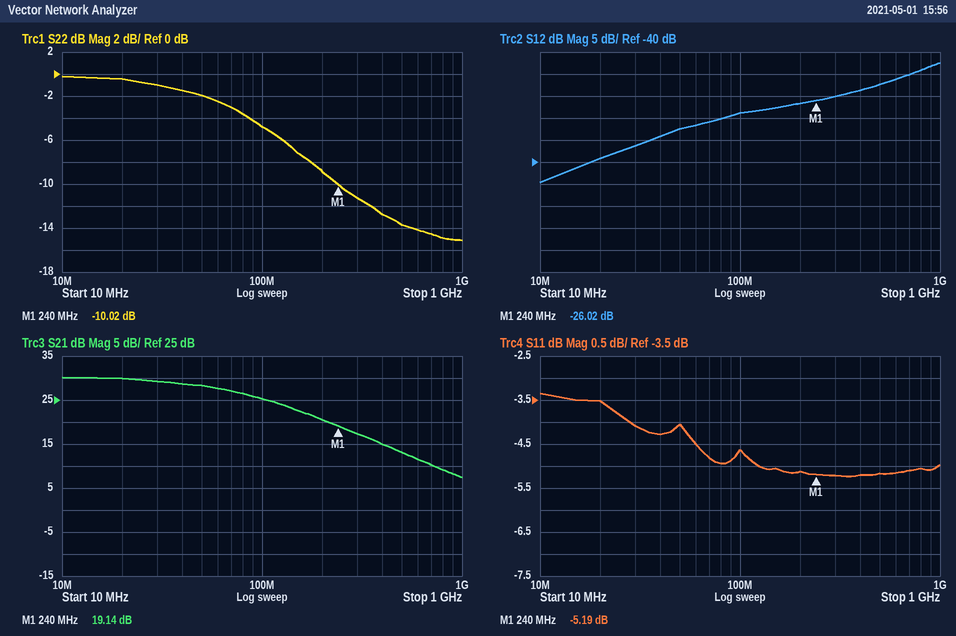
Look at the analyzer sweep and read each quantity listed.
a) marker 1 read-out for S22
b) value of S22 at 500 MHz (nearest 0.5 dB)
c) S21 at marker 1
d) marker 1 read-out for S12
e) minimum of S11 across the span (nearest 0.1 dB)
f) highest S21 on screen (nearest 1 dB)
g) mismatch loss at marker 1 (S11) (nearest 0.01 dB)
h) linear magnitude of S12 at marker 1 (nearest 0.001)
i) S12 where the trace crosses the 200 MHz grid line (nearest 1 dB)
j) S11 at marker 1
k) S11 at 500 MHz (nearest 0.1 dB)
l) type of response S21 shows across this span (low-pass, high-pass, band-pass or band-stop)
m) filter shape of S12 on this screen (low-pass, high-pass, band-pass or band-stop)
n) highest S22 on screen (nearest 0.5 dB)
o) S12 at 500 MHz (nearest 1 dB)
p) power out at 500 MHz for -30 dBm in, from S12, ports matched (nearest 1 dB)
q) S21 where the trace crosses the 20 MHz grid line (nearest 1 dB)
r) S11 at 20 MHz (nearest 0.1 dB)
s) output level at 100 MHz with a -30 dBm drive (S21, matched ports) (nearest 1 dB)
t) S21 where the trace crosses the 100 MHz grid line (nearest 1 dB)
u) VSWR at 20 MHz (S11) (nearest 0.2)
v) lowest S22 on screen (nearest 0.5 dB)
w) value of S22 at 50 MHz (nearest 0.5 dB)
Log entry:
-10.02 dB
-13.5 dB
19.14 dB
-26.02 dB
-5.2 dB
30 dB
1.57 dB
0.050
-27 dB
-5.19 dB
-5.2 dB
low-pass
high-pass
0.0 dB
-22 dB
-52 dBm
30 dB
-3.5 dB
-5 dBm
25 dB
5.0
-15.0 dB
-2.0 dB
